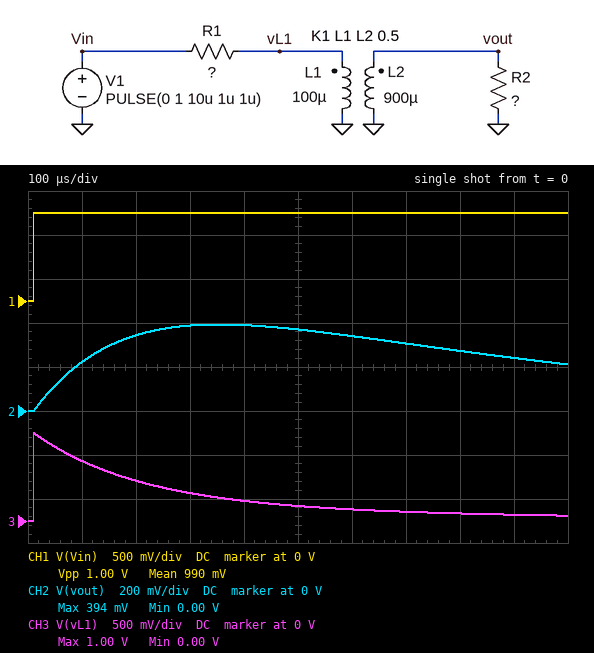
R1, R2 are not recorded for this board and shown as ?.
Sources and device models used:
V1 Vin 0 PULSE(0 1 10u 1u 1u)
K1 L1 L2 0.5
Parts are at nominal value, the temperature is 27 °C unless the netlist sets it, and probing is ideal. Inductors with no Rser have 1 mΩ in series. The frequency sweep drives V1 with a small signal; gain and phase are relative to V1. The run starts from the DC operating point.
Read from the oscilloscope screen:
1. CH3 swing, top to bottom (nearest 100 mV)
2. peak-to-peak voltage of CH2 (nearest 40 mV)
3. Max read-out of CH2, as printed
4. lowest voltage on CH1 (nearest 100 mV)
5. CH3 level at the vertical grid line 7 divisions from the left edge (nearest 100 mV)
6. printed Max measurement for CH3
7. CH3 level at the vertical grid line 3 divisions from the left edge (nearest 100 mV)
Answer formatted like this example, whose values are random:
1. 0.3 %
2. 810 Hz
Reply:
1. 1.0 V
2. 400 mV
3. 394 mV
4. 0 V
5. 100 mV
6. 1.00 V
7. 300 mV
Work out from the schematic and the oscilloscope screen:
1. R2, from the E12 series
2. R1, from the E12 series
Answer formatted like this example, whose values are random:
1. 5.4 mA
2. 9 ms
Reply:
1. 1.5 Ω
2. 0.33 Ω
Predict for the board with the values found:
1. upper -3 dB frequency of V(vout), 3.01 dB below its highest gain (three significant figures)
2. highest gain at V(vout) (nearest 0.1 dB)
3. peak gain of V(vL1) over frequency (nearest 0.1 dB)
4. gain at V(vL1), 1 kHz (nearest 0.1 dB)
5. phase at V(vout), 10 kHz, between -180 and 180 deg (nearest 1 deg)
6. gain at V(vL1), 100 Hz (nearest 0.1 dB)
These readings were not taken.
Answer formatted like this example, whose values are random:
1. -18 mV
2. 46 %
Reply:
1. 1.21 kHz
2. -6.0 dB
3. 0 dB
4. -2.0 dB
5. -84 deg
6. -14.9 dB
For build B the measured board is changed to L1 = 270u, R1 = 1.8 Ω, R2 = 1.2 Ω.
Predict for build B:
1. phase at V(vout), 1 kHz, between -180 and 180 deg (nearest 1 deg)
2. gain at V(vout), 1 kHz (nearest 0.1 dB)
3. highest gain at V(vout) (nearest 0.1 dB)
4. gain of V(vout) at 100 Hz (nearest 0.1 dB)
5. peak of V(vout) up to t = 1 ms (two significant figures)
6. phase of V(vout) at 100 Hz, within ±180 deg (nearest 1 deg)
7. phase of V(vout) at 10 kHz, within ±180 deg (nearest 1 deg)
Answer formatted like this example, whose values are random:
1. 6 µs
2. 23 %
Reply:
1. -22 deg
2. -17.0 dB
3. -16.4 dB
4. -22.3 dB
5. 130 mV
6. 60 deg
7. -80 deg
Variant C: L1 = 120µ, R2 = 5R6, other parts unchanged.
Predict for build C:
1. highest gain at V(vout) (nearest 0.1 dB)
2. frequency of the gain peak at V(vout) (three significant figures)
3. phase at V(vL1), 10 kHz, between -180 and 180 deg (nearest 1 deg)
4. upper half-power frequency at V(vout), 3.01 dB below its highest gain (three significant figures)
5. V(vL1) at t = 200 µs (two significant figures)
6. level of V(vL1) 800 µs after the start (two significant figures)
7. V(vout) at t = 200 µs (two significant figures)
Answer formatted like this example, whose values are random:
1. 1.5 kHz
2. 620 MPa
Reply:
1. -0.5 dB
2. 761 Hz
3. 3 deg
4. 2.17 kHz
5. 550 mV
6. 130 mV
7. 750 mV
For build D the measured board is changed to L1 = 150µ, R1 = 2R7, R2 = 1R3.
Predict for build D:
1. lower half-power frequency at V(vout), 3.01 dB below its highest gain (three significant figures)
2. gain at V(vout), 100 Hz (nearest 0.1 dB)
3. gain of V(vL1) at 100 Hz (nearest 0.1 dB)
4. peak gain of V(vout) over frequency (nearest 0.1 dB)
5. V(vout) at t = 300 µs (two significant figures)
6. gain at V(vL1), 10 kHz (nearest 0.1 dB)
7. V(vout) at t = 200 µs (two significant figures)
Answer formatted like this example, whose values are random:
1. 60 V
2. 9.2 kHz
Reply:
1. 203 Hz
2. -28.2 dB
3. -29.5 dB
4. -20.8 dB
5. 68 mV
6. -0.6 dB
7. 77 mV
